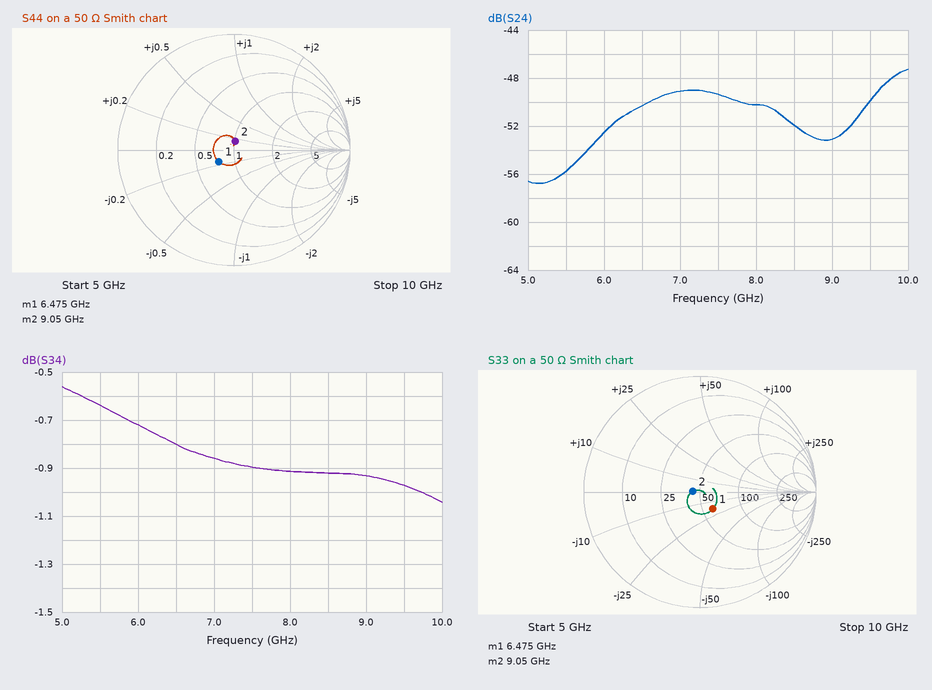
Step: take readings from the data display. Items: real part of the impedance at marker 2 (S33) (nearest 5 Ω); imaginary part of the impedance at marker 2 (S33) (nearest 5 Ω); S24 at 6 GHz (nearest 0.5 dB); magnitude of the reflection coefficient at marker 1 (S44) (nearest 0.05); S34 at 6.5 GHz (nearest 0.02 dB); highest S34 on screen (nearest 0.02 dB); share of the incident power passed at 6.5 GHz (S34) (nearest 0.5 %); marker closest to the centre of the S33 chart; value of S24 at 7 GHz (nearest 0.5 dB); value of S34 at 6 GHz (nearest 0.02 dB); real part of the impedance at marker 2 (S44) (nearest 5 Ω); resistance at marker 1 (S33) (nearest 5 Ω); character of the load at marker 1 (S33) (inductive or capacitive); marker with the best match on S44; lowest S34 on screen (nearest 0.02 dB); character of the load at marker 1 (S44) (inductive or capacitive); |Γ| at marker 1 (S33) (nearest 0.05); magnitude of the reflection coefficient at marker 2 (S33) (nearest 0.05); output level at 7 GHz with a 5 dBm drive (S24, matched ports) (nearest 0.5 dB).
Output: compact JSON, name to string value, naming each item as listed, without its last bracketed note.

{"real part of the impedance at marker 2 (S33)": "45 Ω", "imaginary part of the impedance at marker 2 (S33)": "0 Ω", "S24 at 6 GHz": "-52.5 dB", "magnitude of the reflection coefficient at marker 1 (S44)": "0.15", "S34 at 6.5 GHz": "-0.80 dB", "highest S34 on screen": "-0.56 dB", "share of the incident power passed at 6.5 GHz (S34)": "83.0 %", "marker closest to the centre of the S33 chart": "marker 2", "value of S24 at 7 GHz": "-49.0 dB", "value of S34 at 6 GHz": "-0.72 dB", "real part of the impedance at marker 2 (S44)": "50 Ω", "resistance at marker 1 (S33)": "60 Ω", "character of the load at marker 1 (S33)": "capacitive", "marker with the best match on S44": "marker 2", "lowest S34 on screen": "-1.04 dB", "character of the load at marker 1 (S44)": "capacitive", "|Γ| at marker 1 (S33)": "0.20", "magnitude of the reflection coefficient at marker 2 (S33)": "0.05", "output level at 7 GHz with a 5 dBm drive (S24, matched ports)": "-44.0 dBm"}
